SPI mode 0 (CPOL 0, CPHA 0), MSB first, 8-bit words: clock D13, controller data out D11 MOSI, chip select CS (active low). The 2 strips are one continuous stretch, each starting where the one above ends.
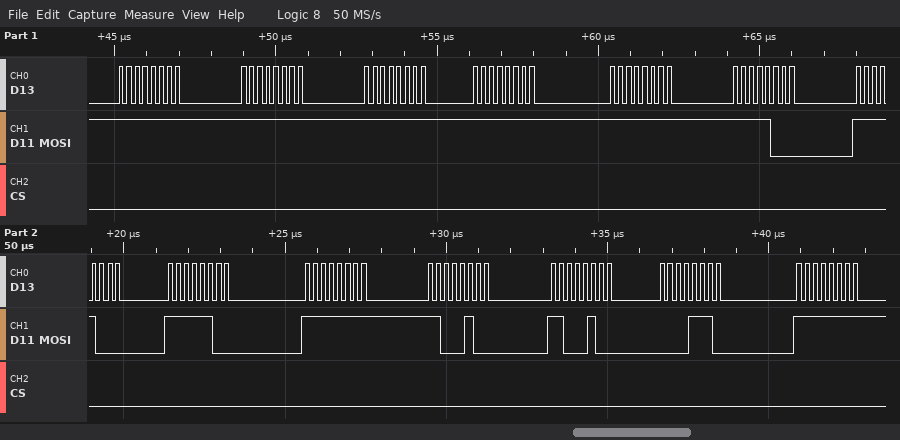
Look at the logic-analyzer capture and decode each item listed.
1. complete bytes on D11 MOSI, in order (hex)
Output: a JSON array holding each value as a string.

["0xFF 0xFF 0xFF 0xFF 0xFF 0xF8 0xF8 0xFC 0xFF 0xC4 0xC4 0x0E 0xFF"]
